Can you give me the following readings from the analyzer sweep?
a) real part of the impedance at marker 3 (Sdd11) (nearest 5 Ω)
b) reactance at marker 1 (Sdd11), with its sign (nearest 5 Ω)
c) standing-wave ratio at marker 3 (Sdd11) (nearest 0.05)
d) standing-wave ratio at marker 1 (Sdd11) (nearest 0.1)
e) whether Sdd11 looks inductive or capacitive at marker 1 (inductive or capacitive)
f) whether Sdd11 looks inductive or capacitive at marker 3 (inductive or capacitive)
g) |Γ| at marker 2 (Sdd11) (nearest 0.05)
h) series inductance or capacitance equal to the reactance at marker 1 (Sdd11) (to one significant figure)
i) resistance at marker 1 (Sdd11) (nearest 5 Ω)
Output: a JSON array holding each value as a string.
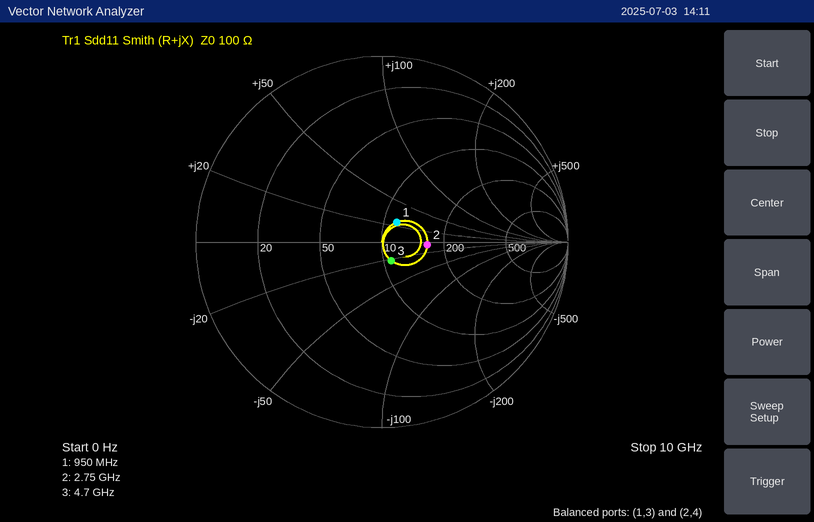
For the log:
["110 Ω", "+25 Ω", "1.25", "1.3", "inductive", "capacitive", "0.25", "4 nH", "115 Ω"]
